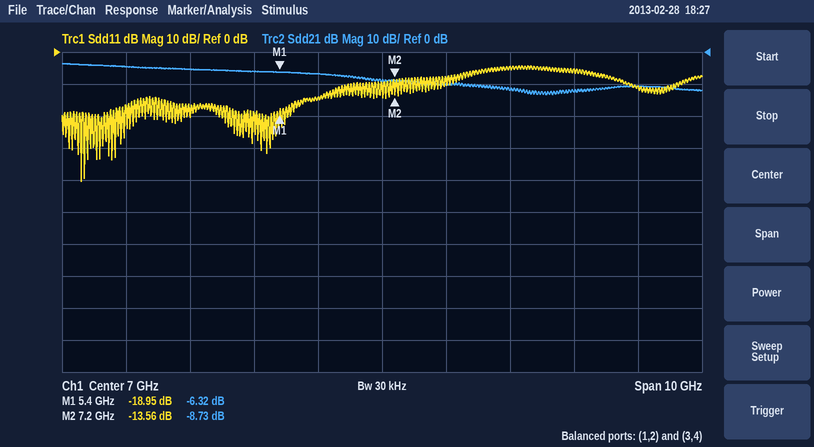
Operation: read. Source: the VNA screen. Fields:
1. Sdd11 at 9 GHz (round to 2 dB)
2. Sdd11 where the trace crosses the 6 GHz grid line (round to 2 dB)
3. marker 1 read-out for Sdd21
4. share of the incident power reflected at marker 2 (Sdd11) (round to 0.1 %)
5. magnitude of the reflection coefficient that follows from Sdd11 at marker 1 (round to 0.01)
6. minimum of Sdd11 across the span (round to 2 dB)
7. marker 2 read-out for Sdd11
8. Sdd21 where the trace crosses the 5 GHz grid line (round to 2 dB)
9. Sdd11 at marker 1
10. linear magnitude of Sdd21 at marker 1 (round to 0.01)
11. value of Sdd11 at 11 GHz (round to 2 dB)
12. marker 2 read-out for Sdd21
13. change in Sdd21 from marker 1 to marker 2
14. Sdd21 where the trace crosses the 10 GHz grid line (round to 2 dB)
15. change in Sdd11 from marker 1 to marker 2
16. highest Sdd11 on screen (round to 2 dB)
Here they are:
-4 dB
-14 dB
-6.32 dB
4.4 %
0.11
-40 dB
-13.56 dB
-6 dB
-18.95 dB
0.48
-10 dB
-8.73 dB
-2.41 dB
-12 dB
5.39 dB
-4 dB
